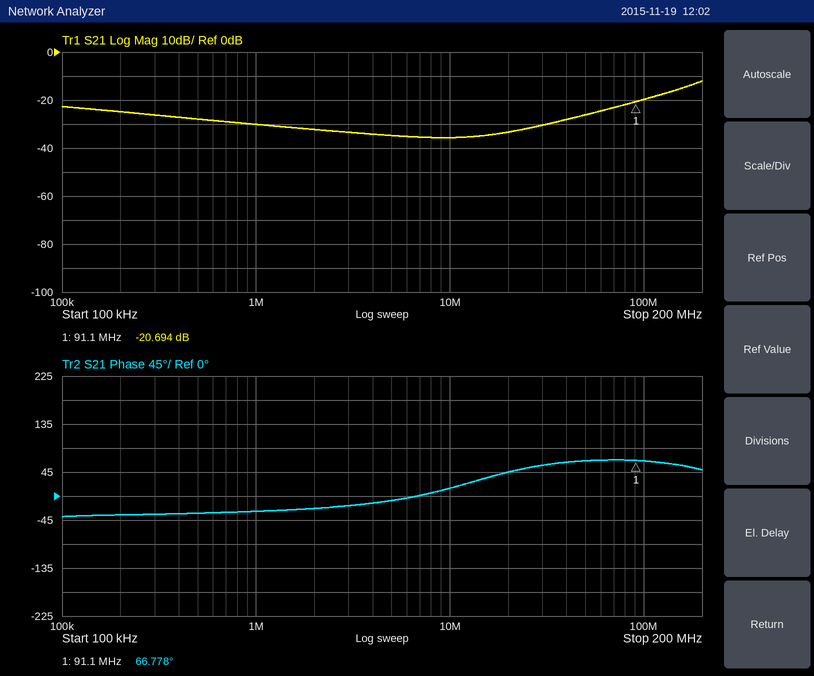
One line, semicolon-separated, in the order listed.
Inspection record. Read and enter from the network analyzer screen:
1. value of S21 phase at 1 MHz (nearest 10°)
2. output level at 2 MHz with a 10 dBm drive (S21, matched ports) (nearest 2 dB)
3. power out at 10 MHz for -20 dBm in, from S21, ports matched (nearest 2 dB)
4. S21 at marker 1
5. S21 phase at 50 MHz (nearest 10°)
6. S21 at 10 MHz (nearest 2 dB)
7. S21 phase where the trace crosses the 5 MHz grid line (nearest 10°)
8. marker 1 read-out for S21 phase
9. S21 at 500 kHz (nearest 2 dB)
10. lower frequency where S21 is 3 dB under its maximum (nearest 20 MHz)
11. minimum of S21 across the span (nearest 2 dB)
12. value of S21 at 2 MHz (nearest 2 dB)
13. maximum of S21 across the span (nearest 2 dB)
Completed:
-30°; -22 dBm; -56 dBm; -20.694 dB; 70°; -36 dB; -10°; 66.778°; -28 dB; 160 MHz; -36 dB; -32 dB; -12 dB
